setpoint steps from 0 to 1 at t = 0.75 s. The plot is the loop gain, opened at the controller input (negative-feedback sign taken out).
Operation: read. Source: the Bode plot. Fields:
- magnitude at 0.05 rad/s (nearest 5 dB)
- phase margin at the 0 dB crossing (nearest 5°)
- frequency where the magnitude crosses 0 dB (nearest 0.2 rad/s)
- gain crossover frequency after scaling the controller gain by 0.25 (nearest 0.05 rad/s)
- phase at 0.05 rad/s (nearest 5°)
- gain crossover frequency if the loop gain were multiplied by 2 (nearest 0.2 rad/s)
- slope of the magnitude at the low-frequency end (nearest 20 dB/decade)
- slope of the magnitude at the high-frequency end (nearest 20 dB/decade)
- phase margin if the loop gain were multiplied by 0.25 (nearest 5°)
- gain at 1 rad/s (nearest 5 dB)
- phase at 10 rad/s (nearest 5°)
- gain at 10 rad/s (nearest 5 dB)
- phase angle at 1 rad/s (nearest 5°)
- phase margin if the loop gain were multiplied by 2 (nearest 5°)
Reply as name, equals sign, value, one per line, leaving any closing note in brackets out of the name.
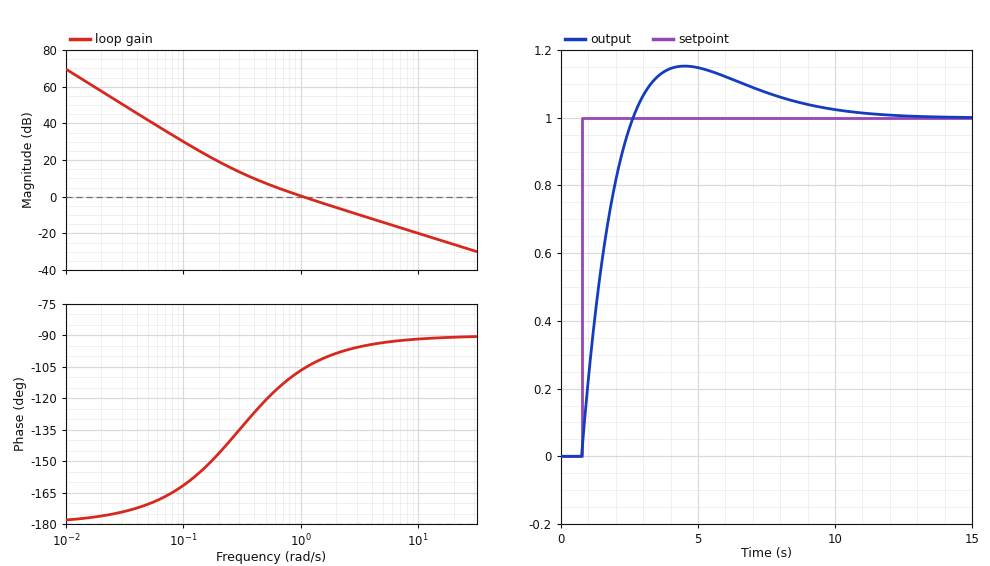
magnitude at 0.05 rad/s = 40 dB
phase margin at the 0 dB crossing = 75°
frequency where the magnitude crosses 0 dB = 1.0 rad/s
gain crossover frequency after scaling the controller gain by 0.25 = 0.35 rad/s
phase at 0.05 rad/s = -170°
gain crossover frequency if the loop gain were multiplied by 2 = 2.0 rad/s
slope of the magnitude at the low-frequency end = -40 dB/decade
slope of the magnitude at the high-frequency end = -20 dB/decade
phase margin if the loop gain were multiplied by 0.25 = 50°
gain at 1 rad/s = 0 dB
phase at 10 rad/s = -90°
gain at 10 rad/s = -20 dB
phase angle at 1 rad/s = -105°
phase margin if the loop gain were multiplied by 2 = 80°
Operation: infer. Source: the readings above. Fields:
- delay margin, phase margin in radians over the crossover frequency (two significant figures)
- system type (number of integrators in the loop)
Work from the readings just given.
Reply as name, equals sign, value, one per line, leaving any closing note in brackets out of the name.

delay margin, phase margin in radians over the crossover frequency = 1.3 s
system type = 2
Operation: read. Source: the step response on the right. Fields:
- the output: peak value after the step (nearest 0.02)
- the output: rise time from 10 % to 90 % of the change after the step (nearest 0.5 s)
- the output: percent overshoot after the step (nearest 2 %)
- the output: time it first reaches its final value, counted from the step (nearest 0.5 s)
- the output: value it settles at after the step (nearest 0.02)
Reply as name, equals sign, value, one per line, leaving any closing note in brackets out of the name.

the output: peak value after the step = 1.16
the output: rise time from 10 % to 90 % of the change after the step = 1.5 s
the output: percent overshoot after the step = 16 %
the output: time it first reaches its final value, counted from the step = 2.0 s
the output: value it settles at after the step = 1.00
